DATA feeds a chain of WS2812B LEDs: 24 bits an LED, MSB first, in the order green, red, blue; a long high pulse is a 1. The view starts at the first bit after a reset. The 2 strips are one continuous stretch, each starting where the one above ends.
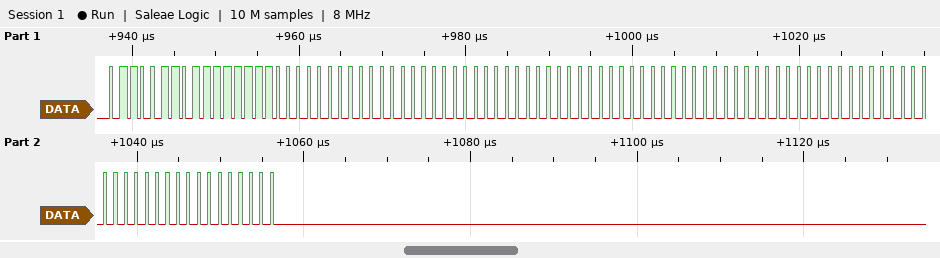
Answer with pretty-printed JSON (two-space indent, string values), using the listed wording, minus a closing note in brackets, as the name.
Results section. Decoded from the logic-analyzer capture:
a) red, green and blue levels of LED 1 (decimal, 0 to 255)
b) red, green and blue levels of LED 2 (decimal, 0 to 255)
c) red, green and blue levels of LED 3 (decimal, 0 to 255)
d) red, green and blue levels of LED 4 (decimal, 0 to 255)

{
  "red, green and blue levels of LED 1": "255, 102, 0",
  "red, green and blue levels of LED 2": "0, 0, 0",
  "red, green and blue levels of LED 3": "0, 0, 0",
  "red, green and blue levels of LED 4": "0, 0, 0"
}
